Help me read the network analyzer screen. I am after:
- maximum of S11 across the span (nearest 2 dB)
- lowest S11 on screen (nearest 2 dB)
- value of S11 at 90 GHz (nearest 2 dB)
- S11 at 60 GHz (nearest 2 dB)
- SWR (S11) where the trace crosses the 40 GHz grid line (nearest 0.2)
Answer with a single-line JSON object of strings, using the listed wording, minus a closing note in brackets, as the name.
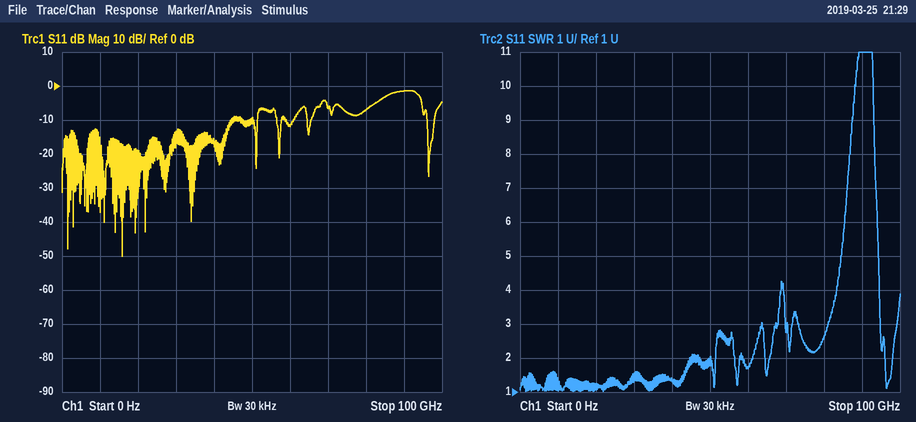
{"maximum of S11 across the span": "-2 dB", "lowest S11 on screen": "-50 dB", "value of S11 at 90 GHz": "-2 dB", "S11 at 60 GHz": "-12 dB", "SWR (S11) where the trace crosses the 40 GHz grid line": "1.4"}
